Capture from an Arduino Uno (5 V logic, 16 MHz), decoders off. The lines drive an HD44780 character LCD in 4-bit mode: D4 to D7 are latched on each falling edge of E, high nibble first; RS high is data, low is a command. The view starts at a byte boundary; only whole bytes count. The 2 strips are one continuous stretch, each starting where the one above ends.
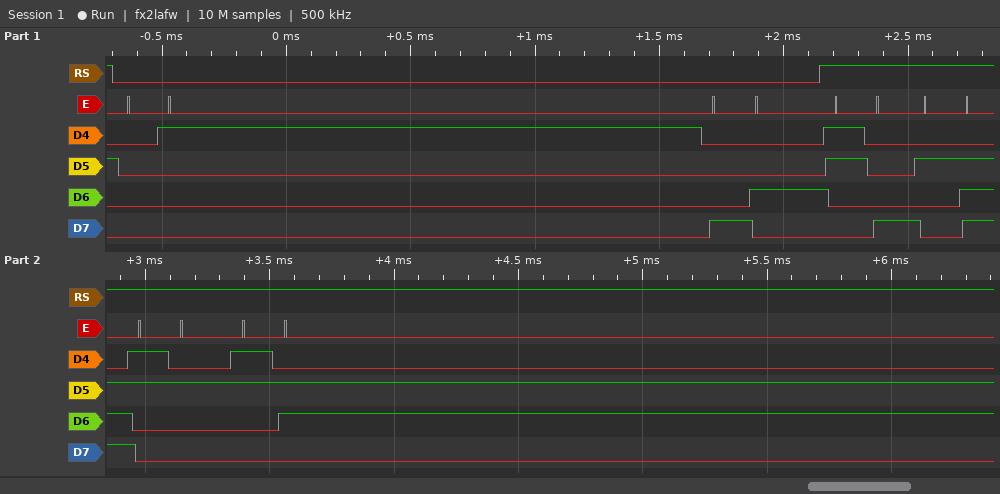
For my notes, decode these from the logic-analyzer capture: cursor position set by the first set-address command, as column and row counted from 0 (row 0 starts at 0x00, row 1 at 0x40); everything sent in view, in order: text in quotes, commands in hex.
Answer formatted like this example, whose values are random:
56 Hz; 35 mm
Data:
column 4, row 0; 0x01 0x84 "8.26"
